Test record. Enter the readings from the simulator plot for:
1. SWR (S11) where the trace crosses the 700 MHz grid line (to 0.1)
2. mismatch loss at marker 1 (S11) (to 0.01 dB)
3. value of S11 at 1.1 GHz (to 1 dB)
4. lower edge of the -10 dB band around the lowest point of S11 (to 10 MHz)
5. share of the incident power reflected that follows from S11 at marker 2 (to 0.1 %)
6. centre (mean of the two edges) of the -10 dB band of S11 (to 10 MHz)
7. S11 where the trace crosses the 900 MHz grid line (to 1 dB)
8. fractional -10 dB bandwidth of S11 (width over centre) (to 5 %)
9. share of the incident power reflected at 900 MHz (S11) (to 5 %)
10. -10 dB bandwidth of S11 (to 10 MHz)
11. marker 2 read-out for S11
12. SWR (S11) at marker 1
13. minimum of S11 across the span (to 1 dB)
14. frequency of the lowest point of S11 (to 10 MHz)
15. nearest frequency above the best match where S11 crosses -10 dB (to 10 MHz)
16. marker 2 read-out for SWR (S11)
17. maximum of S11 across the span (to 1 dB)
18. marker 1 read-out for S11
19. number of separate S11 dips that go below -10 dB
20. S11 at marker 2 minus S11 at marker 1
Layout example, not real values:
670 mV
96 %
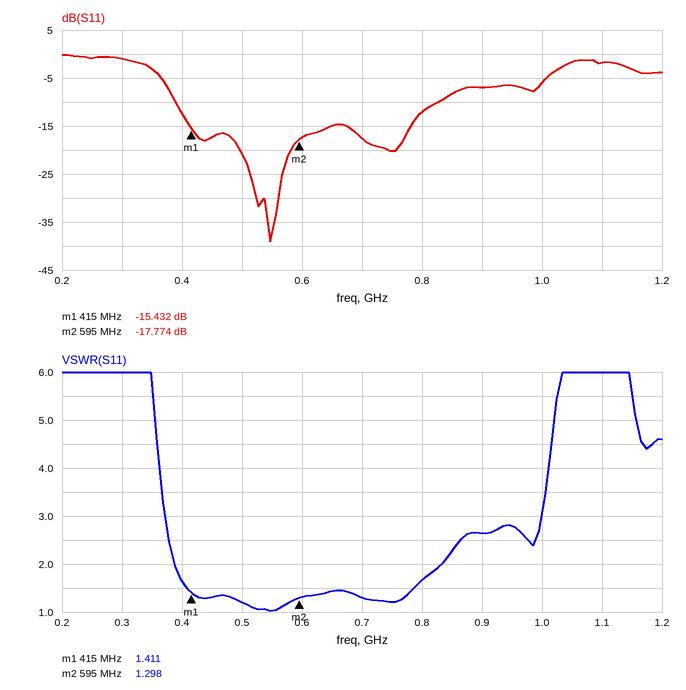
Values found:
1.3
0.13 dB
-2 dB
390 MHz
1.7 %
610 MHz
-7 dB
70 %
20 %
440 MHz
-17.774 dB
1.411
-39 dB
550 MHz
830 MHz
1.298
0 dB
-15.432 dB
2
-2.342 dB
